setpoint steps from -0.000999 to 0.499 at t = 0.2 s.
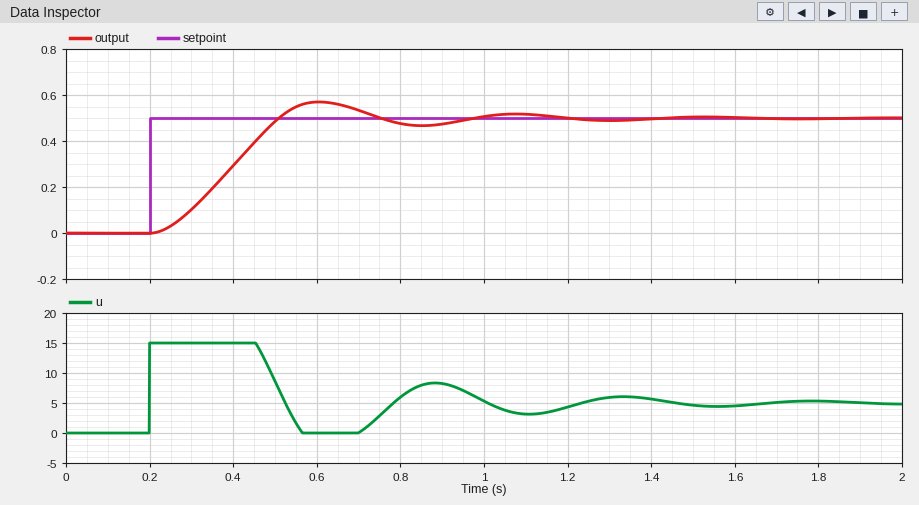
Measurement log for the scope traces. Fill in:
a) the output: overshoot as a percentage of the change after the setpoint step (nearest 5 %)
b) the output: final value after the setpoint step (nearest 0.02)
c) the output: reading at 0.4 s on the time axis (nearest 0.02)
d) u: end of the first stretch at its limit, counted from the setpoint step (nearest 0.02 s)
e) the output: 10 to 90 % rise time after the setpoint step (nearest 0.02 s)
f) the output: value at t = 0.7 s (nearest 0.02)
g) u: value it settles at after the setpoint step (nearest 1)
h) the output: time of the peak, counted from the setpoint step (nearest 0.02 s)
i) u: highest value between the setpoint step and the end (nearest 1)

15 %
0.50
0.30
0.26 s
0.22 s
0.54
5
0.40 s
15
